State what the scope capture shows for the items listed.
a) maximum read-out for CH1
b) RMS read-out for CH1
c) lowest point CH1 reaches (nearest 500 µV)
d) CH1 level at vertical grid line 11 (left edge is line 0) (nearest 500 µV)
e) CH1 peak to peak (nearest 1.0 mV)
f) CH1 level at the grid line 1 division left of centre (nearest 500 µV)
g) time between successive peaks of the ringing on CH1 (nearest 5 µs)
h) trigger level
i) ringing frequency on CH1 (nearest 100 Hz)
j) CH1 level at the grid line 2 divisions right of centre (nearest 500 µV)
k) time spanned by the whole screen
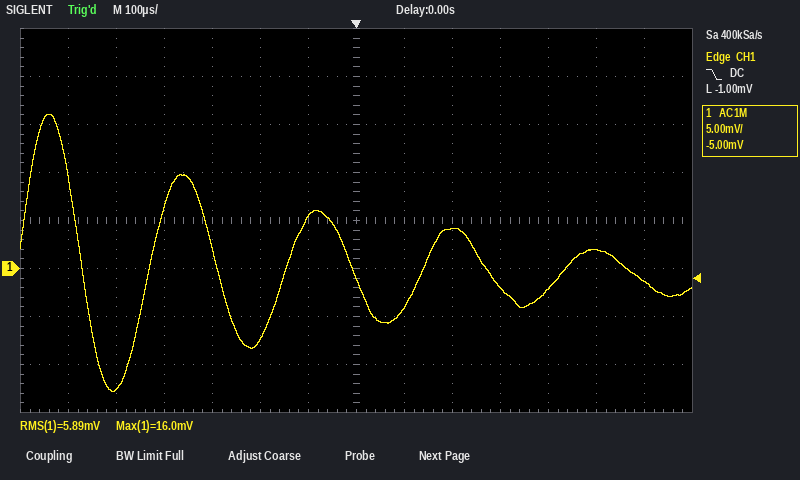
16.0 mV
5.89 mV
-13.0 mV
-2.0 mV
29.0 mV
5.5 mV
285 µs
-1.00 mV
3.5 kHz
4.0 mV
1.4 ms
